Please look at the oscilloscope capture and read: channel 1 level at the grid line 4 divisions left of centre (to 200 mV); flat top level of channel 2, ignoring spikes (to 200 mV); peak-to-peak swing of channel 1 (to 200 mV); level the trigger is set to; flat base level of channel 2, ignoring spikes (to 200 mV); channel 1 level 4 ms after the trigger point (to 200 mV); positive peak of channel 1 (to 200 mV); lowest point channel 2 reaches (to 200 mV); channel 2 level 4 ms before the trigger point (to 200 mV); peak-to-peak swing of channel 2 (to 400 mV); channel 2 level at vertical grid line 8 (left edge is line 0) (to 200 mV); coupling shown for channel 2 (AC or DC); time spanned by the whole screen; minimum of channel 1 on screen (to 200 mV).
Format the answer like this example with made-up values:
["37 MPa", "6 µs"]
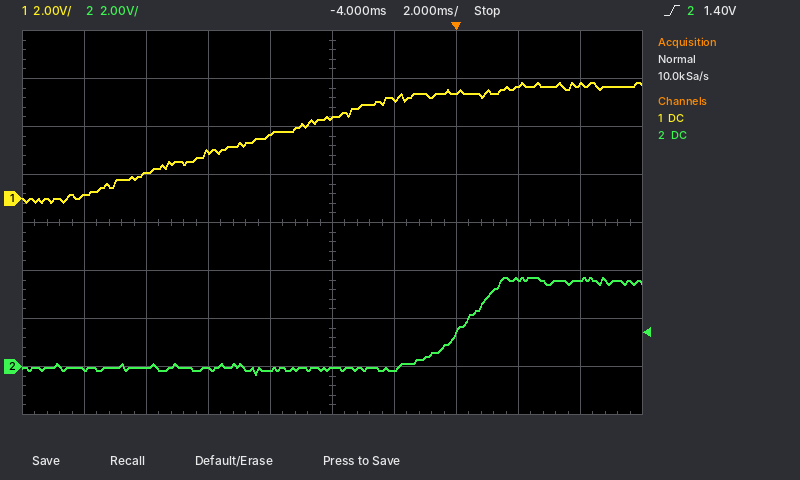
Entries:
["200 mV", "3.6 V", "5.0 V", "1.40 V", "0.0 V", "4.8 V", "4.8 V", "-400 mV", "0.0 V", "4.0 V", "3.6 V", "DC", "20 ms", "-200 mV"]
